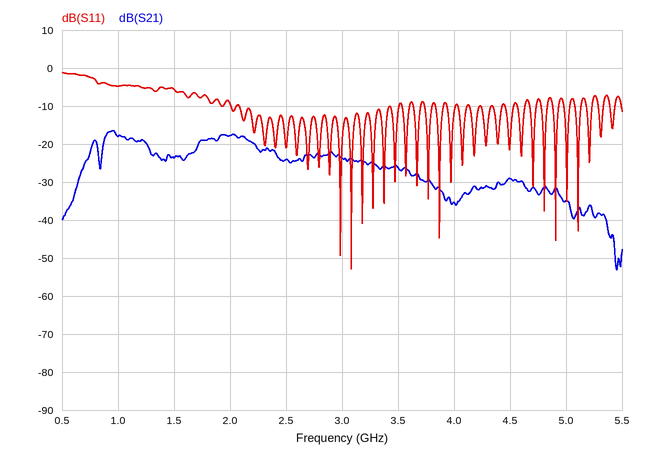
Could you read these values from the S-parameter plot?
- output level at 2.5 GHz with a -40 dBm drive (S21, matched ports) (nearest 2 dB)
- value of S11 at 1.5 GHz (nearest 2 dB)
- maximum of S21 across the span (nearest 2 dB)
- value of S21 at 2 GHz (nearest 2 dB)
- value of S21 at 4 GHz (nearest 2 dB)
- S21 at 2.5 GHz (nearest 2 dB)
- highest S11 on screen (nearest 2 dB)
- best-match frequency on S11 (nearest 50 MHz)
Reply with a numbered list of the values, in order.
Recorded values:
1. -64 dBm
2. -6 dB
3. -16 dB
4. -18 dB
5. -36 dB
6. -24 dB
7. -2 dB
8. 3.10 GHz
